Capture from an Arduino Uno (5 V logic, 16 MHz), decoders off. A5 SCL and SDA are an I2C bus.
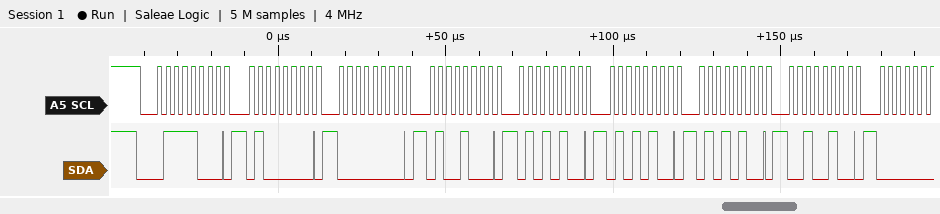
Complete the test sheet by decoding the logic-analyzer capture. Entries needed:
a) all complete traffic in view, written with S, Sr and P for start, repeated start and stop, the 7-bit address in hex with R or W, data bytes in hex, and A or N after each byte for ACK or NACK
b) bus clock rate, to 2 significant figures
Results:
S 3CW A 40 A 00 A 48 A 54 A 54 A 54 A 24 A
400 kHz
